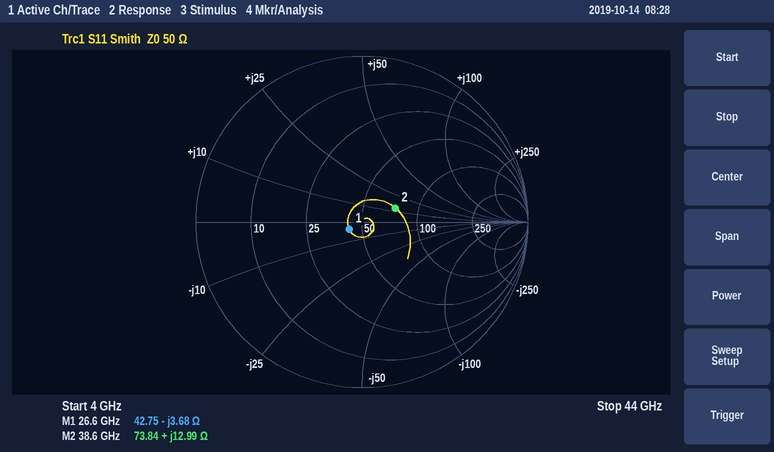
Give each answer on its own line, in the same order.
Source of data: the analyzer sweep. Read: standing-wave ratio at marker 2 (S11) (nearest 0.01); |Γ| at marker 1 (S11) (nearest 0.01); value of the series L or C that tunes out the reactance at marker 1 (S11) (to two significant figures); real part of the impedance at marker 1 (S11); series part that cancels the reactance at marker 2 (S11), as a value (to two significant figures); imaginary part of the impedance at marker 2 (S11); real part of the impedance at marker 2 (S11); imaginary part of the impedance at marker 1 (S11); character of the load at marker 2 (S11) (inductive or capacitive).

1.56
0.09
22 pH
42.75 Ω
320 fF
+12.99 Ω
73.84 Ω
-3.68 Ω
inductive
